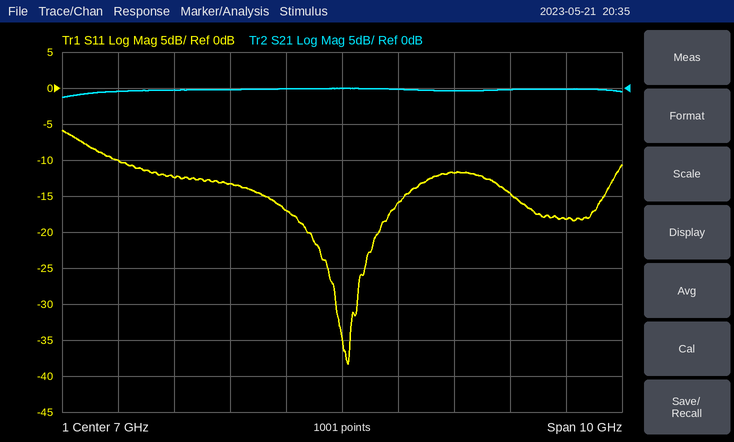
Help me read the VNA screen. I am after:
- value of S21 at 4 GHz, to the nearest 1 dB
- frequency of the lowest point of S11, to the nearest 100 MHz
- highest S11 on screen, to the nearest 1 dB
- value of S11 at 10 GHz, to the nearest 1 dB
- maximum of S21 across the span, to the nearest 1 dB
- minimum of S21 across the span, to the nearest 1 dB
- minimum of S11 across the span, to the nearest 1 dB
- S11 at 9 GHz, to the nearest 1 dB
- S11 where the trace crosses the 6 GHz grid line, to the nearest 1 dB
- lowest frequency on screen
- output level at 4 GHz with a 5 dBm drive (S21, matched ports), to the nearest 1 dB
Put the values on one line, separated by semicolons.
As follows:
0 dB; 7.1 GHz; -6 dB; -15 dB; 0 dB; -1 dB; -38 dB; -12 dB; -17 dB; 2 GHz; 5 dBm
